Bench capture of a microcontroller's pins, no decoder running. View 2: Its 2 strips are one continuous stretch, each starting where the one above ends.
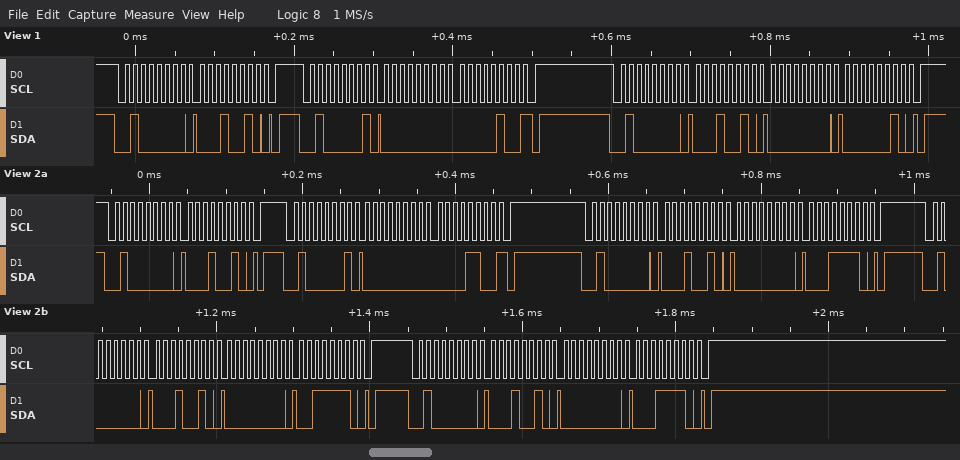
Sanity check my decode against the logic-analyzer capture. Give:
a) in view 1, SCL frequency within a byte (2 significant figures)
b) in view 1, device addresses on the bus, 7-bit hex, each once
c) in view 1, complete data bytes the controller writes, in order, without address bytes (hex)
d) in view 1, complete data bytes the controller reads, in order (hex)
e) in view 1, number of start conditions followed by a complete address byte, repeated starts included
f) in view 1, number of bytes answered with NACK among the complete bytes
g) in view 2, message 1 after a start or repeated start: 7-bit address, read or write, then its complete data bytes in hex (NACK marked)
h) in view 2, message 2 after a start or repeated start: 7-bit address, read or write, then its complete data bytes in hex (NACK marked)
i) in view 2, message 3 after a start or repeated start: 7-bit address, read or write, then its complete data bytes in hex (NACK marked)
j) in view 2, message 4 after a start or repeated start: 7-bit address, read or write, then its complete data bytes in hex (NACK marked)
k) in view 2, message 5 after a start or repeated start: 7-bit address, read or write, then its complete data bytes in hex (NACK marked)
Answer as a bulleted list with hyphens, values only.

- 100 kHz
- 0x20
- 12 12 00 02
- 00 04
- 3
- 1
- 0x20 write: 12
- 0x20 read: 00 0C NACK
- 0x20 write: 12 00 1E
- 0x20 write: 12 00 3E
- 0x20 write: 12 00 1E
